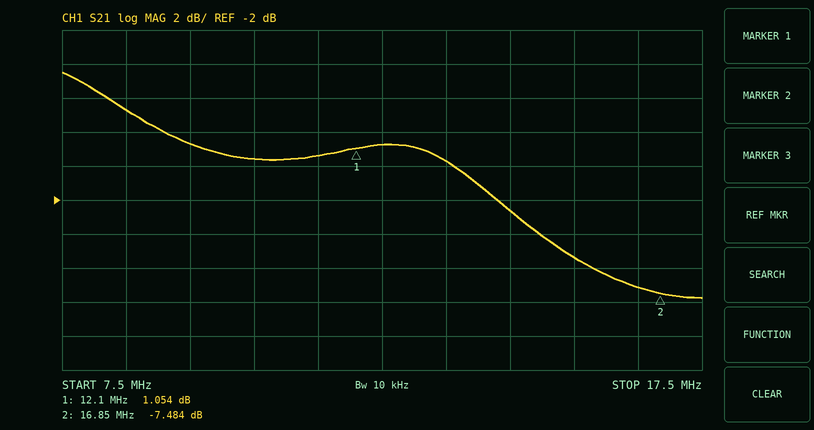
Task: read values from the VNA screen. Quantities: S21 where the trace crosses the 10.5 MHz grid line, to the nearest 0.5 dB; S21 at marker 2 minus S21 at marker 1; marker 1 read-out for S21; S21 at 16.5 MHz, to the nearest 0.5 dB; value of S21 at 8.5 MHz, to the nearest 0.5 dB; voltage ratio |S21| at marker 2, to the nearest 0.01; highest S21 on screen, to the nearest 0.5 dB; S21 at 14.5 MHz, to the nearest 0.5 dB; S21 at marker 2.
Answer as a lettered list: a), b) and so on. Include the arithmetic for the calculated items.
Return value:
a) 0.5 dB
b) -7.484 − (1.054) = -8.538 dB
c) 1.054 dB
d) -7.0 dB
e) 3.5 dB
f) 10^(-7.484/20) ≈ 0.42
g) 5.5 dB
h) -2.5 dB
i) -7.484 dB
